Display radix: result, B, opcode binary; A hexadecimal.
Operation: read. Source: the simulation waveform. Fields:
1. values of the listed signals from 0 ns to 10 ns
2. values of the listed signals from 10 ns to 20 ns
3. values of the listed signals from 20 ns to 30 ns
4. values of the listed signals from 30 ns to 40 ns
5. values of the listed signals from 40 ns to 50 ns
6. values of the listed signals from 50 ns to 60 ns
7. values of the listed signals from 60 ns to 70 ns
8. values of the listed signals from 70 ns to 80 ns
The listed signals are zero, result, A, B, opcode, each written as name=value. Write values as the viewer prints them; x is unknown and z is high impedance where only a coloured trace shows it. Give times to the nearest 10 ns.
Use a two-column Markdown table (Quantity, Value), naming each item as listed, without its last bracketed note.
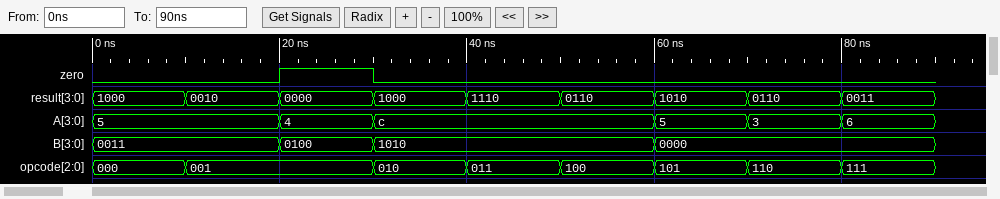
| Quantity | Value |
|---|---|
| values of the listed signals from 0 ns to 10 ns | zero=0, result=1000, A=5, B=0011, opcode=000 |
| values of the listed signals from 10 ns to 20 ns | zero=0, result=0010, A=5, B=0011, opcode=001 |
| values of the listed signals from 20 ns to 30 ns | zero=1, result=0000, A=4, B=0100, opcode=001 |
| values of the listed signals from 30 ns to 40 ns | zero=0, result=1000, A=c, B=1010, opcode=010 |
| values of the listed signals from 40 ns to 50 ns | zero=0, result=1110, A=c, B=1010, opcode=011 |
| values of the listed signals from 50 ns to 60 ns | zero=0, result=0110, A=c, B=1010, opcode=100 |
| values of the listed signals from 60 ns to 70 ns | zero=0, result=1010, A=5, B=0000, opcode=101 |
| values of the listed signals from 70 ns to 80 ns | zero=0, result=0110, A=3, B=0000, opcode=110 |
